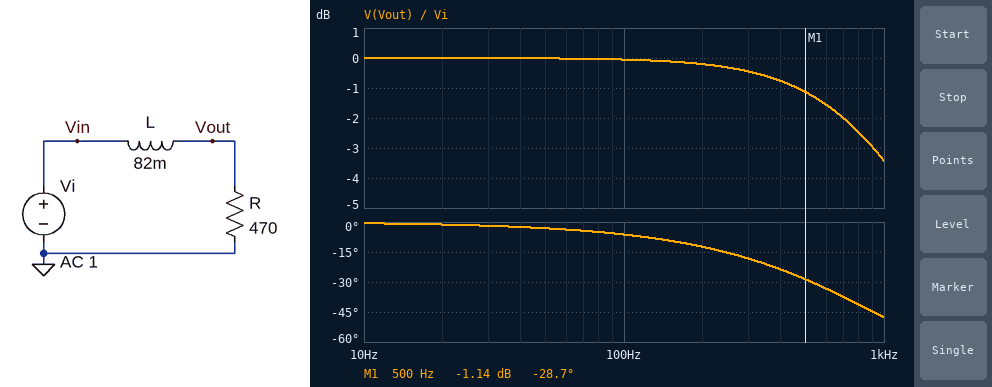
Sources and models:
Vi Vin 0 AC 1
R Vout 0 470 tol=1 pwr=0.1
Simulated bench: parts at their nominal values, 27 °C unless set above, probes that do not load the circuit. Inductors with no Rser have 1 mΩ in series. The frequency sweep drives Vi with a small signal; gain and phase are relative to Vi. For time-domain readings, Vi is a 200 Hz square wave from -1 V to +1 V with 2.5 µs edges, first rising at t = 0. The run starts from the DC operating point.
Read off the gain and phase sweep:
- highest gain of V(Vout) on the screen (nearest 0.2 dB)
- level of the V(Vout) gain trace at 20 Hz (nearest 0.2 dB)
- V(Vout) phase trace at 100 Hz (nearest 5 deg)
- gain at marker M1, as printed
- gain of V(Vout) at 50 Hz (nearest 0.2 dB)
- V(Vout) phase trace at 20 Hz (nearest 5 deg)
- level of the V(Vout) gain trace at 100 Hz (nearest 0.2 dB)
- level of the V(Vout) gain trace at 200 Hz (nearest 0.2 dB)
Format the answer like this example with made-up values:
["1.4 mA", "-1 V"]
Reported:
["0 dB", "0 dB", "-5 deg", "-1.14 dB", "0 dB", "0 deg", "0 dB", "-0.2 dB"]
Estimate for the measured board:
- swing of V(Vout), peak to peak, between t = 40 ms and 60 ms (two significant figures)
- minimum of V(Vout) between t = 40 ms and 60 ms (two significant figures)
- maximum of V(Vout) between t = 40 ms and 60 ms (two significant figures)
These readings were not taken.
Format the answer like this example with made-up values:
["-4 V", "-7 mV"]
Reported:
["2.0 V", "-1.0 V", "1.0 V"]
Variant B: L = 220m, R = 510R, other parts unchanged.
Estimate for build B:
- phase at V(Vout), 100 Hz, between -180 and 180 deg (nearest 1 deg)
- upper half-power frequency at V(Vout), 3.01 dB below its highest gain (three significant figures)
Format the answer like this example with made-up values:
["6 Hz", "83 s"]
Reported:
["-15 deg", "369 Hz"]
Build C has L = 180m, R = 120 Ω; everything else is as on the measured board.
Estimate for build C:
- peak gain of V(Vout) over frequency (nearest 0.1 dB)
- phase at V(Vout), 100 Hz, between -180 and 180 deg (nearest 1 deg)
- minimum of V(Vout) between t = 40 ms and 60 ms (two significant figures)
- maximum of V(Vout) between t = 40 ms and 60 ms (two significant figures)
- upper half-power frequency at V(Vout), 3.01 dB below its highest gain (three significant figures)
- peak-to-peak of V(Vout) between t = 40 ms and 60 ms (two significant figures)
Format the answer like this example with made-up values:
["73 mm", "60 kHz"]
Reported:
["0 dB", "-43 deg", "-680 mV", "680 mV", "106 Hz", "1.4 V"]
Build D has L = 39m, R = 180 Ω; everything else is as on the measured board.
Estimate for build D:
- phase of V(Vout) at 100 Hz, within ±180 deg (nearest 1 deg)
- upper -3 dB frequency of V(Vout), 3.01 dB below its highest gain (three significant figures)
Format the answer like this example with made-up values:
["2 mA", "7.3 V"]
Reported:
["-8 deg", "735 Hz"]
